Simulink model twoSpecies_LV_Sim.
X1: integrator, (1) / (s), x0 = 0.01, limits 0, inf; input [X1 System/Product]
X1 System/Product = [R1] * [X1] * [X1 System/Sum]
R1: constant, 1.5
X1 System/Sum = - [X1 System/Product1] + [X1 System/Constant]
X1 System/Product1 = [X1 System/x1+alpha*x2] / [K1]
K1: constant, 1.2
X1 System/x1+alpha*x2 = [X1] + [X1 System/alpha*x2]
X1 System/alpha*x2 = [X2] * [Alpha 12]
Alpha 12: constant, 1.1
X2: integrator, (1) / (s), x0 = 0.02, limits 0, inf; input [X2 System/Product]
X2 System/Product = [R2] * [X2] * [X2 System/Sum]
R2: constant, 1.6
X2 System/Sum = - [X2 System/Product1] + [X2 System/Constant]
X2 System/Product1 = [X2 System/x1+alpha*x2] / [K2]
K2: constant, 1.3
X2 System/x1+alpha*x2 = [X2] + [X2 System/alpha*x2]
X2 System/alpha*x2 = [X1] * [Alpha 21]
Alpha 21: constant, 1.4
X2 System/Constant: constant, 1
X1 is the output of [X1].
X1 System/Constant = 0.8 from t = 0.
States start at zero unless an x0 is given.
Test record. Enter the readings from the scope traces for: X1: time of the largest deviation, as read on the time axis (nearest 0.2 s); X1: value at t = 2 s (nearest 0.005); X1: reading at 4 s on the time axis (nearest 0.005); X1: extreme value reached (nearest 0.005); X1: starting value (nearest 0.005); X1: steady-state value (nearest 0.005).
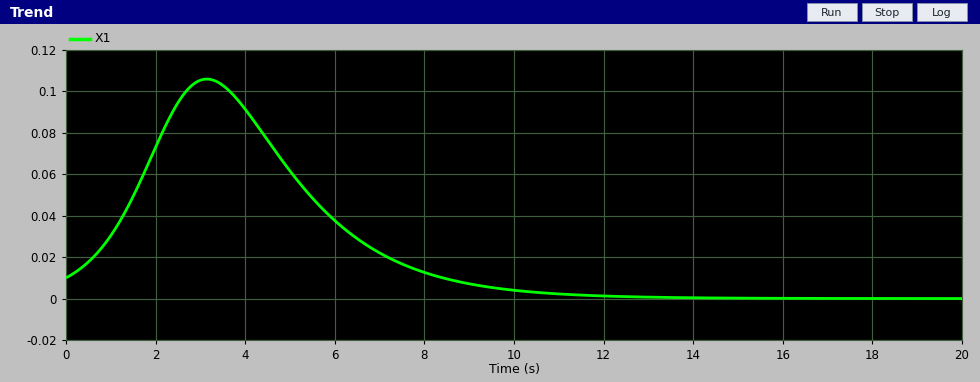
3.2 s
0.075
0.090
0.105
0.010
0.000
